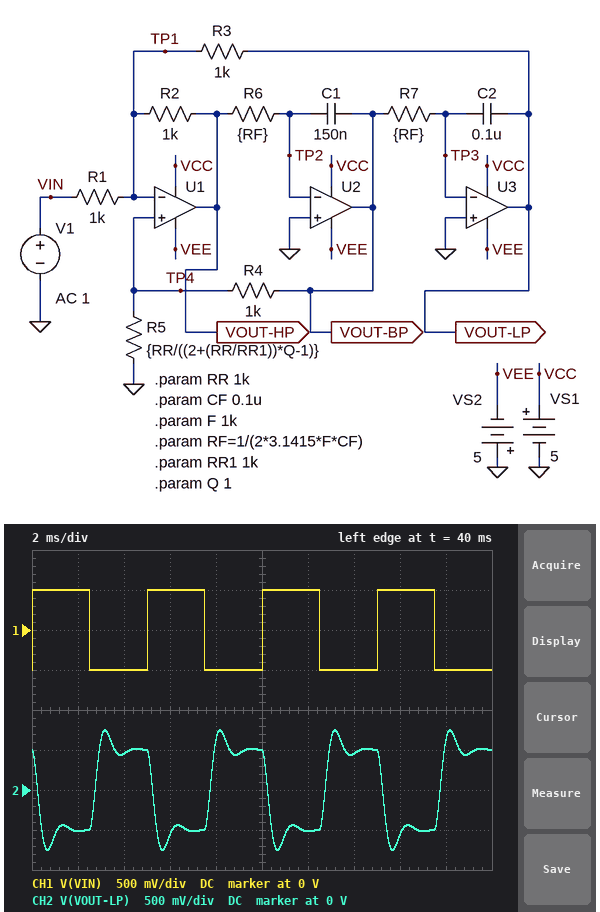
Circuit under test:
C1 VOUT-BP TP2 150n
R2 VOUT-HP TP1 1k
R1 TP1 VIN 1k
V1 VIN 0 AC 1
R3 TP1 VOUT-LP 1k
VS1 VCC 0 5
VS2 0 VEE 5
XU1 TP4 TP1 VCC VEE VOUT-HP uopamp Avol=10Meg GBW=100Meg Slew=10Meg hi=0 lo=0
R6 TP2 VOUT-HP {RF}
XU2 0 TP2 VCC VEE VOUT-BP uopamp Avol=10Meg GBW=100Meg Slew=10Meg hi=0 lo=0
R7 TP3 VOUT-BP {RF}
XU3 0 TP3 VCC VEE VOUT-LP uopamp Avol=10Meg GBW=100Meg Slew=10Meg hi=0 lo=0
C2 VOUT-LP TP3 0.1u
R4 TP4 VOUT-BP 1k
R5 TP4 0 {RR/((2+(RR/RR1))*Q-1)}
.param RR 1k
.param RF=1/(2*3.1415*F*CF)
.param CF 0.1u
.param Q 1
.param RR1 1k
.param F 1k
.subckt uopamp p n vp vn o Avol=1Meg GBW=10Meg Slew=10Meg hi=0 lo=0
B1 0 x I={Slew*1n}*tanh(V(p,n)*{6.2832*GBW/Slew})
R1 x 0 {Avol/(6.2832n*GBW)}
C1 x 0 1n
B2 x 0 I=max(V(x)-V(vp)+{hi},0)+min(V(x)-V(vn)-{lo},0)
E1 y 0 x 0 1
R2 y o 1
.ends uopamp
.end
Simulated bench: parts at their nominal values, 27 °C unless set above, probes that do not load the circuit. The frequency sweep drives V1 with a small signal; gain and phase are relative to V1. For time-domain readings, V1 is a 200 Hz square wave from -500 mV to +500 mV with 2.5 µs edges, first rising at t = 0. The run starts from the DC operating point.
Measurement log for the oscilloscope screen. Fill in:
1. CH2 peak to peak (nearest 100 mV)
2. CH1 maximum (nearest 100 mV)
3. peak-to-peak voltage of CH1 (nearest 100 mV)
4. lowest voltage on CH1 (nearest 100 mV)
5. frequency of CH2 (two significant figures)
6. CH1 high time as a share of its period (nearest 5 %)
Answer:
1.5 V
500 mV
1.0 V
-500 mV
200 Hz
50 %
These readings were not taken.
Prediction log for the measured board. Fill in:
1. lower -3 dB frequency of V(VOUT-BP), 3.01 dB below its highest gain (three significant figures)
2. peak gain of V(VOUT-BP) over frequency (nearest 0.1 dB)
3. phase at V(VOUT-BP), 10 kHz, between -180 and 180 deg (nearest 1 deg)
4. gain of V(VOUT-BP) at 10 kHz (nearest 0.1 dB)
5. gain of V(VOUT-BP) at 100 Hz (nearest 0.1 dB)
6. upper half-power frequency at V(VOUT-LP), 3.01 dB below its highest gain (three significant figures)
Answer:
549 Hz
0 dB
-86 deg
-23.5 dB
-19.9 dB
970 Hz
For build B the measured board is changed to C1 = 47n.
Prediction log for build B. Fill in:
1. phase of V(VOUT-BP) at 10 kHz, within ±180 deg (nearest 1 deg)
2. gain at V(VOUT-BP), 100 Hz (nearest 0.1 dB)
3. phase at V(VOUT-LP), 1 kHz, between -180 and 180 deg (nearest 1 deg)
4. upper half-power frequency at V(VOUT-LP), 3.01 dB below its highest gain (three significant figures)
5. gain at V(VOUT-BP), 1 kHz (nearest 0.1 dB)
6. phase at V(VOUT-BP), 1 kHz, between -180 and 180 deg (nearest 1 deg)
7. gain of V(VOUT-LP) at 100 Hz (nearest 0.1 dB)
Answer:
-78 deg
-20.0 dB
118 deg
1.41 kHz
-1.1 dB
28 deg
0 dB
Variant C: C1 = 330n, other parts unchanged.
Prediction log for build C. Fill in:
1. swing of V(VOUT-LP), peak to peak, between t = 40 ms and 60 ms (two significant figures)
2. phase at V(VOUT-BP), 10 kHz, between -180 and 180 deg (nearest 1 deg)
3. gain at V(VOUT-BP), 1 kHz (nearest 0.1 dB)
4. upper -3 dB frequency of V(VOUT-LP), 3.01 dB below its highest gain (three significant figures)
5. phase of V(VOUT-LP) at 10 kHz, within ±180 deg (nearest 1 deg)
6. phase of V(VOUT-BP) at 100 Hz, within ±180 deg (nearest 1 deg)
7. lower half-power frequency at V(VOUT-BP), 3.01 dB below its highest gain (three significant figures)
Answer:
1.8 V
-88 deg
-8.0 dB
646 Hz
2 deg
84 deg
419 Hz
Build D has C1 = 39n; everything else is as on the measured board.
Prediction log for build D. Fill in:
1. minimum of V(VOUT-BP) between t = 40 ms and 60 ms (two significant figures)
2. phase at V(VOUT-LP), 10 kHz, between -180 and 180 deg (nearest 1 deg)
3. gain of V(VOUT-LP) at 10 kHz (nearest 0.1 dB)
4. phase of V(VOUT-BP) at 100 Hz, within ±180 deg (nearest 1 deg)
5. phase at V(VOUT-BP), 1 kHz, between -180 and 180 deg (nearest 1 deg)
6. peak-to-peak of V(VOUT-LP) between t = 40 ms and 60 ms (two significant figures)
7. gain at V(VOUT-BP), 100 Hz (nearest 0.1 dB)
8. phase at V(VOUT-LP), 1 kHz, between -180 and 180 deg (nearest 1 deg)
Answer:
-680 mV
15 deg
-31.9 dB
84 deg
31 deg
1.0 V
-20.0 dB
121 deg
